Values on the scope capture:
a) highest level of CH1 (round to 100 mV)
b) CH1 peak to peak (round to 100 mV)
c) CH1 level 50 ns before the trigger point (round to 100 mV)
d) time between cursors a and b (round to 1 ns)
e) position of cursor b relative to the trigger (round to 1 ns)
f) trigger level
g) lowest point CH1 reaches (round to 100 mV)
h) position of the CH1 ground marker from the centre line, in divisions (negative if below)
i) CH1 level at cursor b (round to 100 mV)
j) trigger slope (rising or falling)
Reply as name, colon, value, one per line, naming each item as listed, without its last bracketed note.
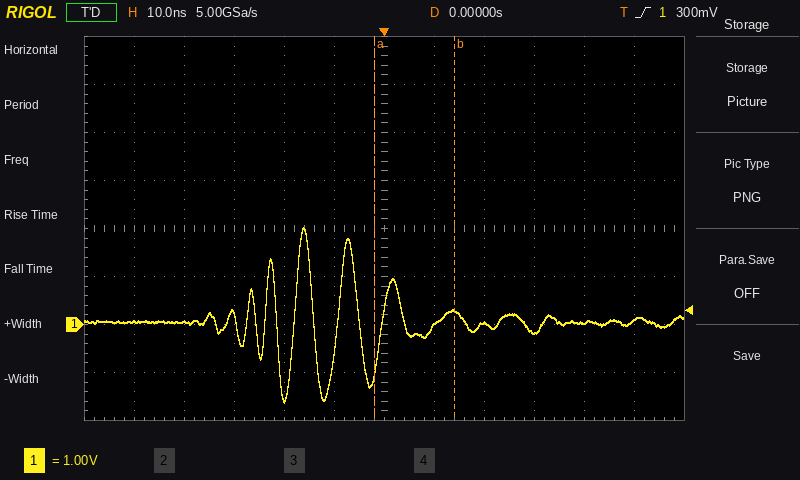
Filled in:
highest level of CH1: 2.0 V
CH1 peak to peak: 3.6 V
CH1 level 50 ns before the trigger point: 100 mV
time between cursors a and b: 16 ns
position of cursor b relative to the trigger: +14 ns
trigger level: 300 mV
lowest point CH1 reaches: -1.6 V
position of the CH1 ground marker from the centre line, in divisions: -2.0 div
CH1 level at cursor b: 300 mV
trigger slope: rising
